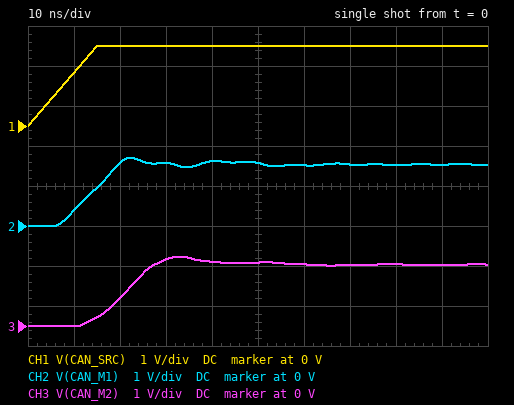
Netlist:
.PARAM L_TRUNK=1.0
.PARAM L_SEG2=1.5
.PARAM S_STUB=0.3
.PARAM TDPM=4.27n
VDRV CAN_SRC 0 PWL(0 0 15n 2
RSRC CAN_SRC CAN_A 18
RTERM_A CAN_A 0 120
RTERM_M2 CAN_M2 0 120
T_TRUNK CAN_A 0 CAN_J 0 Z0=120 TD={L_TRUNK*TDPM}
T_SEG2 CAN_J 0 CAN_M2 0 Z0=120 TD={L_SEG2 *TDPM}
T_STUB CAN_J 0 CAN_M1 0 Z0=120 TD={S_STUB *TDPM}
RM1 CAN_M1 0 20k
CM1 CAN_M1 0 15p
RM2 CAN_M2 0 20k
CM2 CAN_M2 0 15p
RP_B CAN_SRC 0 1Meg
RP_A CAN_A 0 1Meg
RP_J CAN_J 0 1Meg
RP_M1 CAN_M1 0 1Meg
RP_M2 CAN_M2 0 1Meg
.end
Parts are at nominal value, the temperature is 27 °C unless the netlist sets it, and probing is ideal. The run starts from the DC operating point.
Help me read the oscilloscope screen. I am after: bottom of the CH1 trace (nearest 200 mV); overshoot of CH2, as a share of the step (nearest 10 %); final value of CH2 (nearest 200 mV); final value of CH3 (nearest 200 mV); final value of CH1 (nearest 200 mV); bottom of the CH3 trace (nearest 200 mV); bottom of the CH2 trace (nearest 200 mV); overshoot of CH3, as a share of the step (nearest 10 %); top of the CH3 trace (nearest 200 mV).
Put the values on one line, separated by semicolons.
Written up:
0 V; 10 %; 1.6 V; 1.6 V; 2.0 V; 0 V; 0 V; 10 %; 1.8 V
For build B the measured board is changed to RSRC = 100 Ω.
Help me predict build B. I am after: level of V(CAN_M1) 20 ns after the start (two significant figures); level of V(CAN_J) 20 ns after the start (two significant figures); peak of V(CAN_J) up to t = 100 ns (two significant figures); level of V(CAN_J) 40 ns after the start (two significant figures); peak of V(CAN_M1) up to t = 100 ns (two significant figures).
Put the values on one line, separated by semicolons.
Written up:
730 mV; 700 mV; 770 mV; 760 mV; 790 mV
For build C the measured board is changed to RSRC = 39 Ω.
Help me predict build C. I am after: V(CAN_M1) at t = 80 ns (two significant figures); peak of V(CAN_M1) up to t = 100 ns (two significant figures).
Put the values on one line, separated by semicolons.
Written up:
1.2 V; 1.3 V
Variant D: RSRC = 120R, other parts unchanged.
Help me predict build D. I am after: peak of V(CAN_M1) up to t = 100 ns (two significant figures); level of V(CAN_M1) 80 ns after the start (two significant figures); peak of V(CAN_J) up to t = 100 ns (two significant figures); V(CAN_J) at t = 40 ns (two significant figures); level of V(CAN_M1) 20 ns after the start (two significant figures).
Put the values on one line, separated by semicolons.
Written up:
700 mV; 660 mV; 680 mV; 670 mV; 640 mV
